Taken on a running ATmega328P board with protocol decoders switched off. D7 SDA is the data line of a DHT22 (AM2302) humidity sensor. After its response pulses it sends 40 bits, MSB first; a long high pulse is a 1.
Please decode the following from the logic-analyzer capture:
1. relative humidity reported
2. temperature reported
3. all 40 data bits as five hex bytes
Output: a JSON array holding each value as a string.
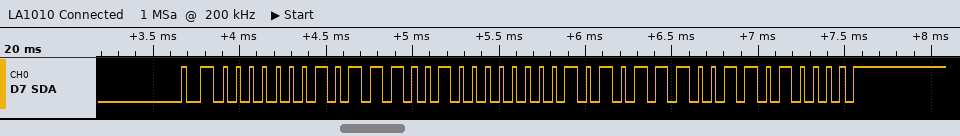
["37.0 %", "34.8 °C", "01 72 01 5C D0"]
